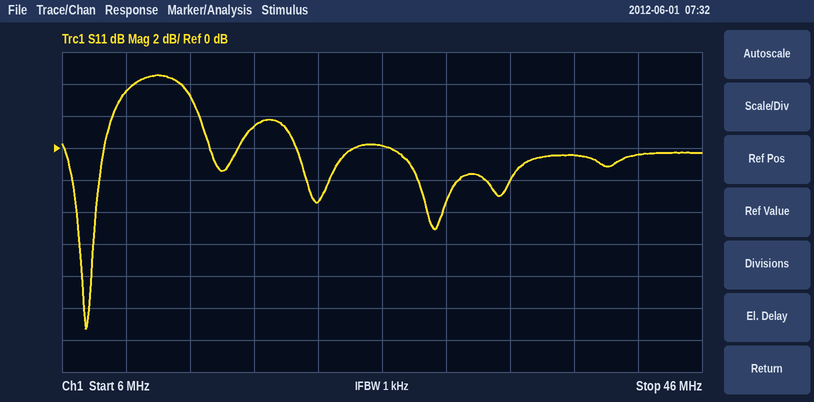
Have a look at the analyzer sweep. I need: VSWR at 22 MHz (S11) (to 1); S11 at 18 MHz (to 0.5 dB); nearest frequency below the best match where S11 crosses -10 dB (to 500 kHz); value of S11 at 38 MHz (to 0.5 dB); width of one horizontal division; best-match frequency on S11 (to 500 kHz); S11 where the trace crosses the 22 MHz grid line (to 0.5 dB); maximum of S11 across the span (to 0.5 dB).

5
1.5 dB
7.5 MHz
-0.5 dB
4 MHz
7.5 MHz
-3.5 dB
4.5 dB
